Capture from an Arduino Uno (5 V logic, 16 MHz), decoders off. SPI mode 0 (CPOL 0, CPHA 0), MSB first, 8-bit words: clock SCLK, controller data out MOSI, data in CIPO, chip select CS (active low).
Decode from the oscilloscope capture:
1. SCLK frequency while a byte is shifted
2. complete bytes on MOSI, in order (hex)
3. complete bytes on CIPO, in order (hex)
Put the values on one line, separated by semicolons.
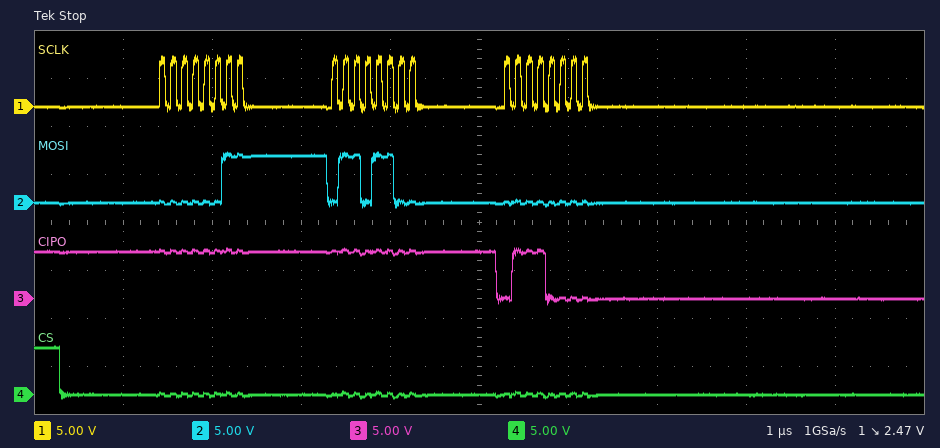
8 MHz; 03 6C 00; FF FF 70
